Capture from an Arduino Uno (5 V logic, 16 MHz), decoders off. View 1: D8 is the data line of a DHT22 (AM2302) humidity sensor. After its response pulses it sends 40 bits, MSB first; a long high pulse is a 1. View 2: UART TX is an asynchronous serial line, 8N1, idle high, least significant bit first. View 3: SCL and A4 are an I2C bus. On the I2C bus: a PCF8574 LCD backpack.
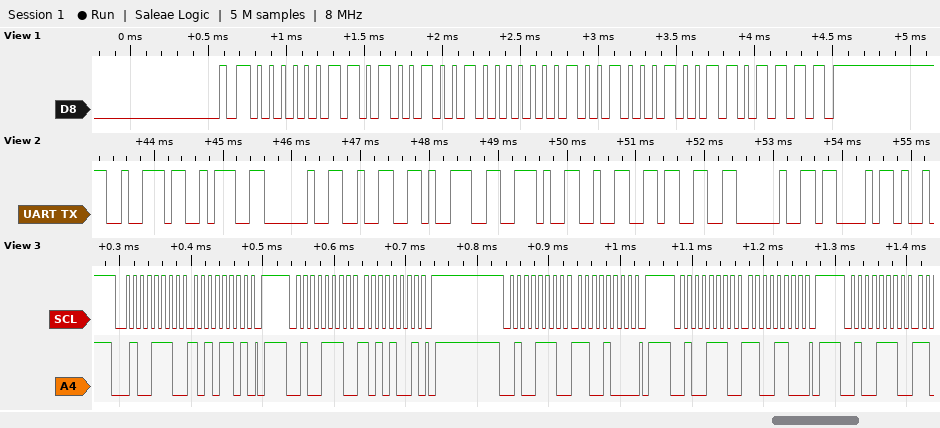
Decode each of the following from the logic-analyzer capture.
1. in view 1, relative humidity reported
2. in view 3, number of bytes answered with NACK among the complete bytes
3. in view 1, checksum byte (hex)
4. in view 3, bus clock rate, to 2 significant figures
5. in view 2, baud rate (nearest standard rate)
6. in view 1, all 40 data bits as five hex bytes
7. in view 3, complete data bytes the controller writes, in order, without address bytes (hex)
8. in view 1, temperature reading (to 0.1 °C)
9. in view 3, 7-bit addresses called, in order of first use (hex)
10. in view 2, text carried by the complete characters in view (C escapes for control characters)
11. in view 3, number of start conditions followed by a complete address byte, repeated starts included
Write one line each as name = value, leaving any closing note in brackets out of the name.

in view 1, relative humidity reported = 84.1 %
in view 3, number of bytes answered with NACK among the complete bytes = 0
in view 1, checksum byte = 0x6F
in view 3, bus clock rate, to 2 significant figures = 100 kHz
in view 2, baud rate = 9600 baud
in view 1, all 40 data bits as five hex bytes = 03 49 01 22 6F
in view 3, complete data bytes the controller writes, in order, without address bytes = AD A9 C8 CC
in view 1, temperature reading = 29.0 °C
in view 3, 7-bit addresses called, in order of first use = 0x27
in view 2, text carried by the complete characters in view = "r: 29.23 C"
in view 3, number of start conditions followed by a complete address byte, repeated starts included = 5
